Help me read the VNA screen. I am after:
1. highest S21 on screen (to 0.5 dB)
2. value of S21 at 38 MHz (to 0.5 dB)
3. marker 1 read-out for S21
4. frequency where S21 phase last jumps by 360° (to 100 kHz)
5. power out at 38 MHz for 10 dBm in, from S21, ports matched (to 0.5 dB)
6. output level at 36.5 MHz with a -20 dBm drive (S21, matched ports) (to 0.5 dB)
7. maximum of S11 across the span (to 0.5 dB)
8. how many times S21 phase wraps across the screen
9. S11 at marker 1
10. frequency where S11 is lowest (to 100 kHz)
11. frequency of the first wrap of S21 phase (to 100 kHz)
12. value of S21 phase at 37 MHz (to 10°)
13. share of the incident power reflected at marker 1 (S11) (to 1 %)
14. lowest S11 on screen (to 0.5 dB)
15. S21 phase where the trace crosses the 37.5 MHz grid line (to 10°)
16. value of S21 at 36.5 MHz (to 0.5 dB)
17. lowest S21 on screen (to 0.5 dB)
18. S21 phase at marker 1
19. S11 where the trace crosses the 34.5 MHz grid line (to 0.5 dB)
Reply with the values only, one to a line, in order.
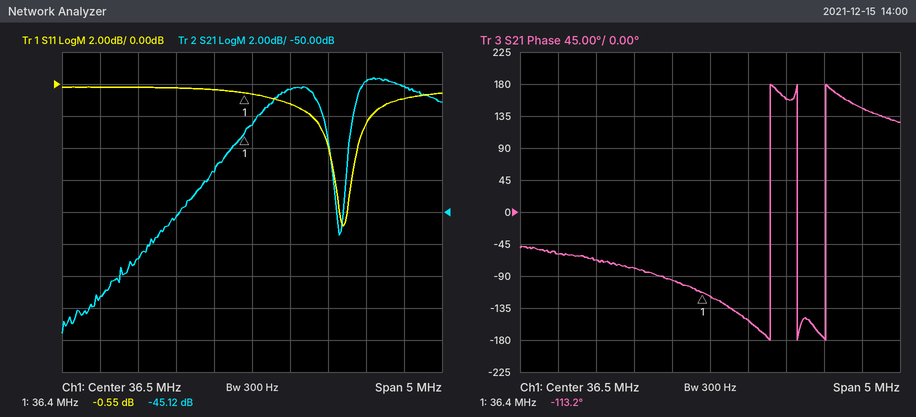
-41.5 dB
-42.0 dB
-45.12 dB
38.0 MHz
-32.0 dBm
-64.5 dBm
0.0 dB
3
-0.55 dB
37.7 MHz
37.3 MHz
-150°
88 %
-9.0 dB
160°
-44.5 dB
-57.5 dB
-113.2°
0.0 dB
